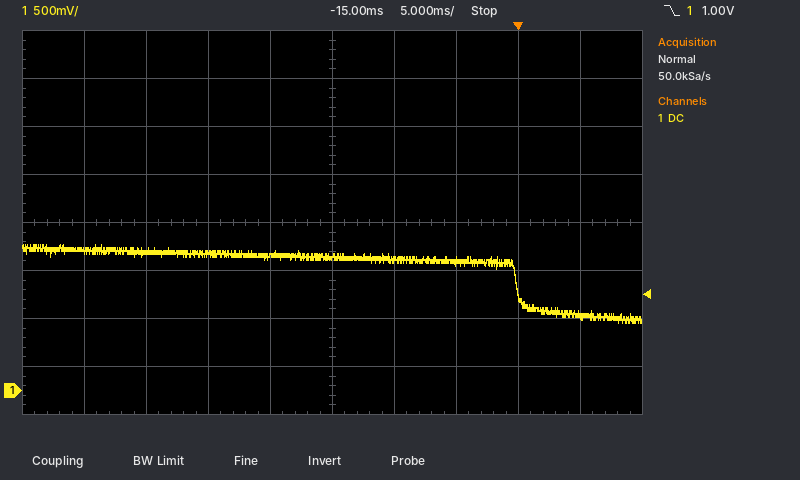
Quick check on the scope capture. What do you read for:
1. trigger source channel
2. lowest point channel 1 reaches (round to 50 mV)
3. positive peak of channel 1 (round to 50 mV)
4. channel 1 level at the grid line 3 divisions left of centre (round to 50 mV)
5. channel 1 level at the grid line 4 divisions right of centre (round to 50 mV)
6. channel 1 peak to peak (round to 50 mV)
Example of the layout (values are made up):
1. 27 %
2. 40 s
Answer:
1. channel 1
2. 700 mV
3. 1.50 V
4. 1.45 V
5. 800 mV
6. 800 mV
